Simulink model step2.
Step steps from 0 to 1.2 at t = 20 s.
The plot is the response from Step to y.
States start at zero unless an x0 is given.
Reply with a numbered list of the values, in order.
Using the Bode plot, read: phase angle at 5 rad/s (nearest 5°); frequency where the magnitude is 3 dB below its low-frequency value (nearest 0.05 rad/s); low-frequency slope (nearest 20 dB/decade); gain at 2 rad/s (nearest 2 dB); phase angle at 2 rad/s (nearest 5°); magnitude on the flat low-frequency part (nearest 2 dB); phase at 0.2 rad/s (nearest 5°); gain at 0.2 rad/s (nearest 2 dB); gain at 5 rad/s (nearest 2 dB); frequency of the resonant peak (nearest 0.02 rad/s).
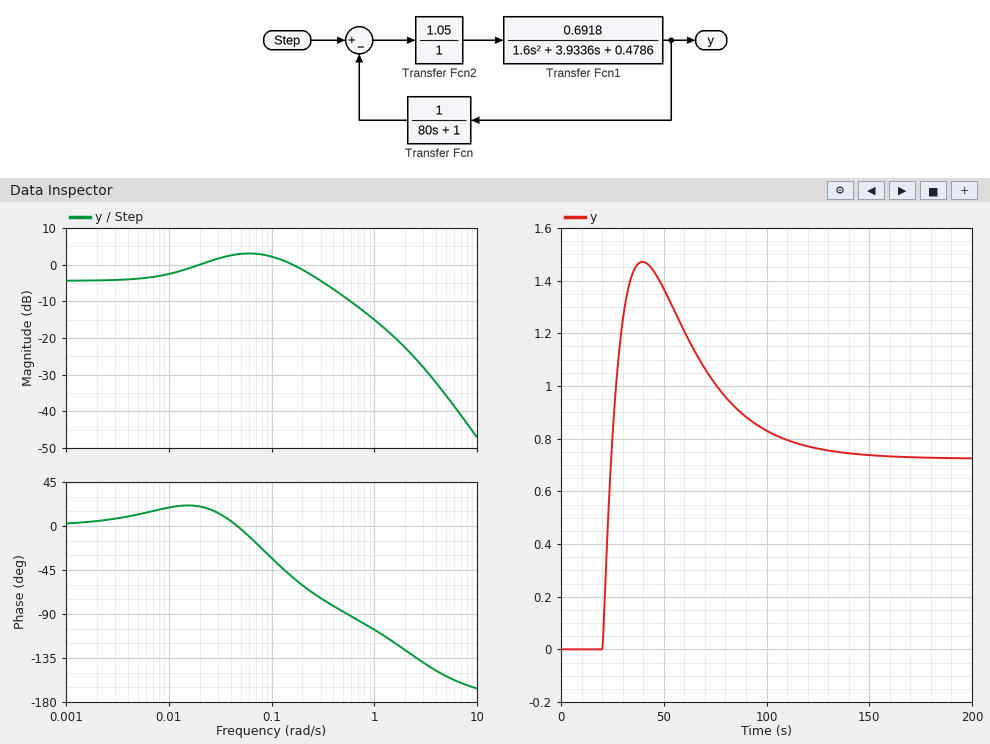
1. -155°
2. 0.45 rad/s
3. 0 dB/decade
4. -22 dB
5. -125°
6. -4 dB
7. -60°
8. -2 dB
9. -36 dB
10. 0.06 rad/s
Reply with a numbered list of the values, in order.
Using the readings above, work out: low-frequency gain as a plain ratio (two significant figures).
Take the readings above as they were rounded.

1. 0.63
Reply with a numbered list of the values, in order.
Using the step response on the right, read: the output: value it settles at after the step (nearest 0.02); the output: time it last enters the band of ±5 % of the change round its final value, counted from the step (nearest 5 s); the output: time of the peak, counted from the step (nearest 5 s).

1. 0.72
2. 105 s
3. 20 s
